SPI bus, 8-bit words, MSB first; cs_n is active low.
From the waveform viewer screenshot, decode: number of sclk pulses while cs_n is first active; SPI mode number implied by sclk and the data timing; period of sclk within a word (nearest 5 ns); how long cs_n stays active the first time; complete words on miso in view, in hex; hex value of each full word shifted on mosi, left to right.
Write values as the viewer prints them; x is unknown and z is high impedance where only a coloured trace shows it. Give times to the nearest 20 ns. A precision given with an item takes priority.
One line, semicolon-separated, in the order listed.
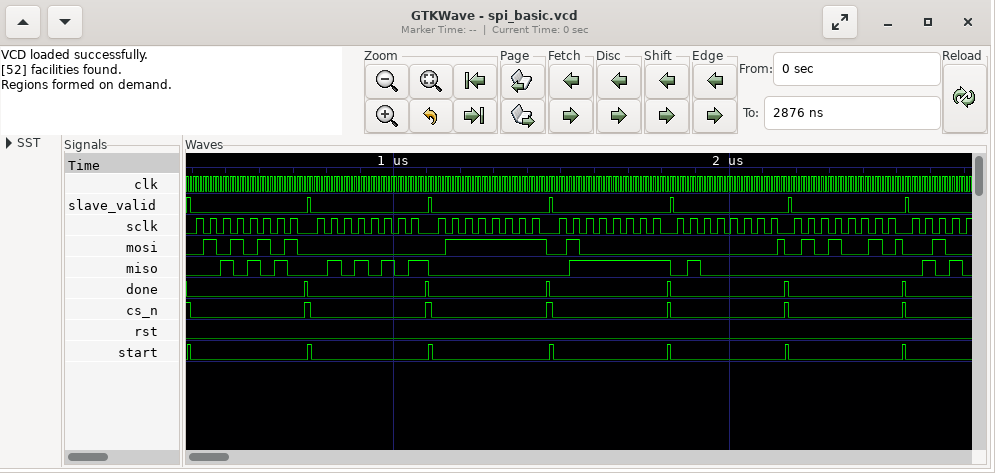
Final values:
8; 0; 40 ns; 340 ns; 2A, 55, 00, 7F, 40, 00; 55, 00, 7F, 40, 00, 52
